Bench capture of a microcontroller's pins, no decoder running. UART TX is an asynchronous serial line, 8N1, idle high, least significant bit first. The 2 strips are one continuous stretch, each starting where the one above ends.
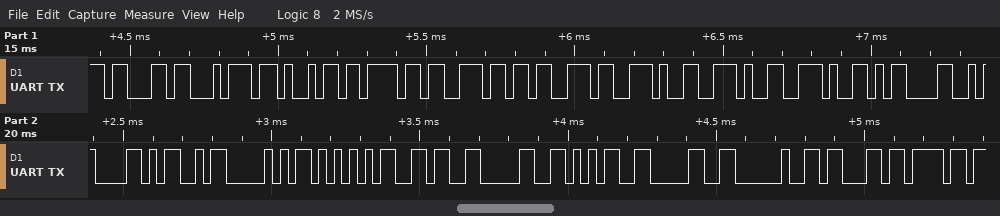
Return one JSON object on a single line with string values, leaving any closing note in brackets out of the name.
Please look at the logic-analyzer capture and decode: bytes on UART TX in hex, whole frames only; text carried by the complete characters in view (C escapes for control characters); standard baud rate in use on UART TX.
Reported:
{"bytes on UART TX in hex, whole frames only": "63 74 69 6F 6E 73 2E 2E 2E 0D 0A 4D 50 55 36 30 35 30 20 63 6F", "text carried by the complete characters in view": "\"ctions...\\r\\nMPU6050 co\"", "standard baud rate in use on UART TX": "38400 baud"}
